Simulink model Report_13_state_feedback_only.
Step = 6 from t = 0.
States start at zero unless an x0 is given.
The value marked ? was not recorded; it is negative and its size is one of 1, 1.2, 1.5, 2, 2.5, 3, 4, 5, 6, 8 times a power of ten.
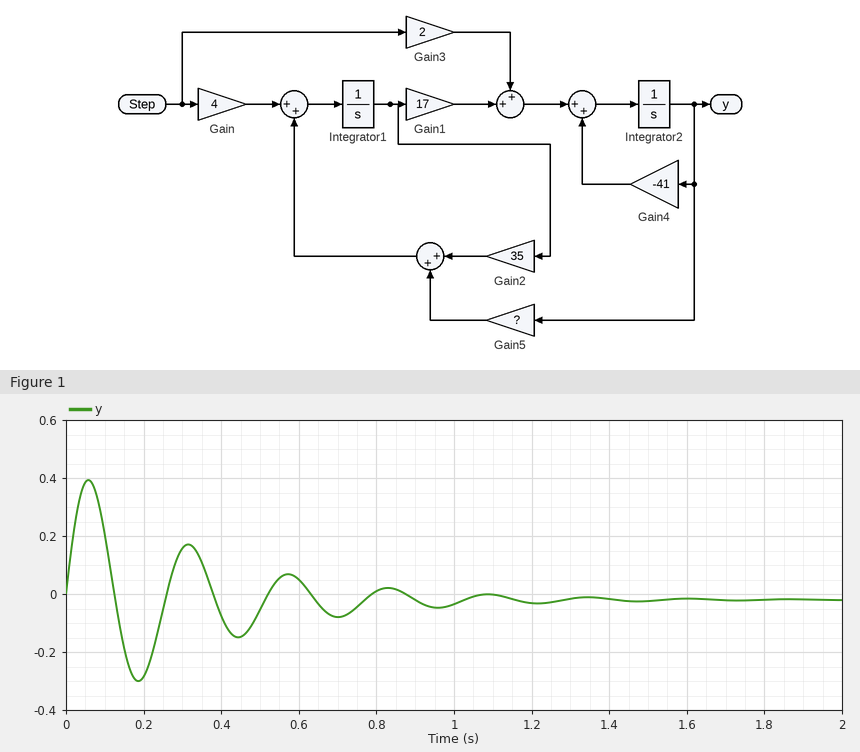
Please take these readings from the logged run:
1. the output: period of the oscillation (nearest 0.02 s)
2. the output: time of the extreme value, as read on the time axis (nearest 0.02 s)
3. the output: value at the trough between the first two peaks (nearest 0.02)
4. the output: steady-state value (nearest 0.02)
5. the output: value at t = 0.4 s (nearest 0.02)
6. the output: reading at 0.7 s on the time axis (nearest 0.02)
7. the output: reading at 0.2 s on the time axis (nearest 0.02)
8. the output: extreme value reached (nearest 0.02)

0.26 s
0.06 s
-0.30
-0.02
-0.08
-0.08
-0.28
0.40
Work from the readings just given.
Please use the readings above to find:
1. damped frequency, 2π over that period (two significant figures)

24 rad/s
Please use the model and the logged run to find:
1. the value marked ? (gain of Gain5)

-120
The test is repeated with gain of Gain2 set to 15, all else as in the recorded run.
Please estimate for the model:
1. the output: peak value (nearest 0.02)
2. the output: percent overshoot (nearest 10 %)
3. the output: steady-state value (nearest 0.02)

0.32
100 %
0.16
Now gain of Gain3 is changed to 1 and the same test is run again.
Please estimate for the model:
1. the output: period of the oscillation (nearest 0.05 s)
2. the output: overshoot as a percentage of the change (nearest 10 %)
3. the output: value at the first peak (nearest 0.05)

0.25 s
90 %
0.60
